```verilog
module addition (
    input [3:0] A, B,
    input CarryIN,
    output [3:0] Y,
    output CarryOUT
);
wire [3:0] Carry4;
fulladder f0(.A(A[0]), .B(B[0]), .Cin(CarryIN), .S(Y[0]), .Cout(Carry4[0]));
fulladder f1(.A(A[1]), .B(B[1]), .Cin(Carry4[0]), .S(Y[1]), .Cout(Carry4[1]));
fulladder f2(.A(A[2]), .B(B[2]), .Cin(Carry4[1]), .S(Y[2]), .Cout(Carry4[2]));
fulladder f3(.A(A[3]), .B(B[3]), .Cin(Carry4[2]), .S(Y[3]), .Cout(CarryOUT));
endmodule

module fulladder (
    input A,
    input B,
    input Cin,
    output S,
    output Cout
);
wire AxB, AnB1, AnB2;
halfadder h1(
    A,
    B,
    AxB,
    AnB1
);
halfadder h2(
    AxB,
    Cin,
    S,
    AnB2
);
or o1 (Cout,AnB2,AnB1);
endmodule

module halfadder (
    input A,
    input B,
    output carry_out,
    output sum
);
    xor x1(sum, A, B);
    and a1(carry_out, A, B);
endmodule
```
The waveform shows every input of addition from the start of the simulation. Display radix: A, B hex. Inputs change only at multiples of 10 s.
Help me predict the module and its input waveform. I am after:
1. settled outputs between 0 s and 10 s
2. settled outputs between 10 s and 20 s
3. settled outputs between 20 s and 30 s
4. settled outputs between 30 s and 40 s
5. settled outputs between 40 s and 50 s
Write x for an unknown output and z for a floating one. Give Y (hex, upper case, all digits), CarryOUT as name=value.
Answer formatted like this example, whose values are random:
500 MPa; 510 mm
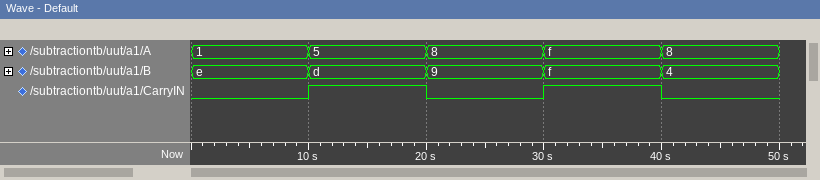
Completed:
Y=0, CarryOUT=1; Y=1, CarryOUT=1; Y=8, CarryOUT=0; Y=5, CarryOUT=1; Y=0, CarryOUT=1
